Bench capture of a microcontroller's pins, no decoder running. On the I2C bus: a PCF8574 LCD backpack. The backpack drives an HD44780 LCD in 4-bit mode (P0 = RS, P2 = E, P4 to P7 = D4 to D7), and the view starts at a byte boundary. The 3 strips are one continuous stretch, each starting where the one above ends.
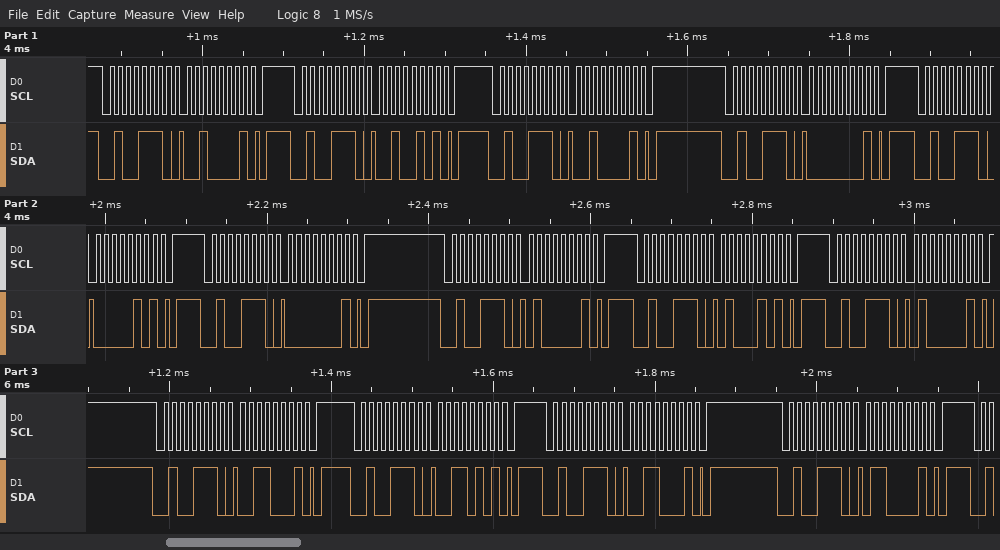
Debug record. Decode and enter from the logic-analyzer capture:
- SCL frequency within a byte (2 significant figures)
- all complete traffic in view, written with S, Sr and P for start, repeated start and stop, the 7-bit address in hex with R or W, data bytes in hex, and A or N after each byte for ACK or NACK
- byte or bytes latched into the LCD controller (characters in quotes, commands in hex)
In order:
100 kHz
S 27W A 21 A P S 27W A 25 A P S 27W A 21 A P S 27W A 01 A P S 27W A 05 A P S 27W A 01 A P S 27W A 41 A P S 27W A 45 A P S 27W A 41 A P S 27W A 31 A P S 27W A 35 A P S 27W A 31 A P S 27W A 61 A P
' ' 'C'
